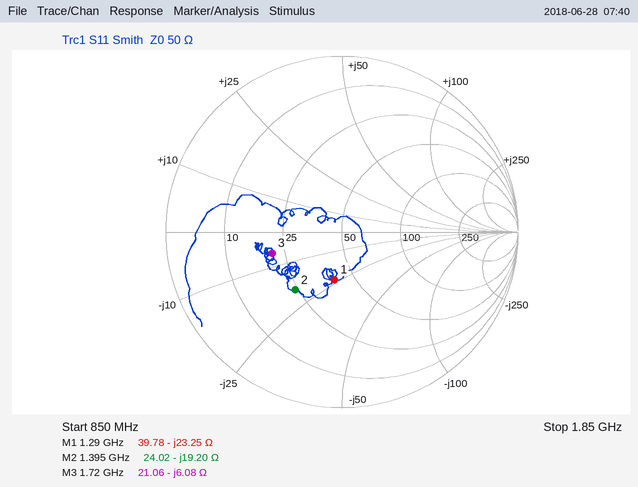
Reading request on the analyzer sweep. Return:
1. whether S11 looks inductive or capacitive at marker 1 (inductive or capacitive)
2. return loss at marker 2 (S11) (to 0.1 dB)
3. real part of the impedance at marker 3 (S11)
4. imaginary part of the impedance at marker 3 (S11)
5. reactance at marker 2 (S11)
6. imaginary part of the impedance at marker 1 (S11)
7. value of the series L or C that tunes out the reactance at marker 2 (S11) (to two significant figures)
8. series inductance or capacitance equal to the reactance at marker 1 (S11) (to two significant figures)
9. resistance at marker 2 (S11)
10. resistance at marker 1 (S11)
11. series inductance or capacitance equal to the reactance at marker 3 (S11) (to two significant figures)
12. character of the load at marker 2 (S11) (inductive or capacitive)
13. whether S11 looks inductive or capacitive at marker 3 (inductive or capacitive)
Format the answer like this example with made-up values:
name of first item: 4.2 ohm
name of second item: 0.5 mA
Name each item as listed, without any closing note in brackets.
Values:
whether S11 looks inductive or capacitive at marker 1: capacitive
return loss at marker 2 (S11): 7.5 dB
real part of the impedance at marker 3: 21.06 Ω
imaginary part of the impedance at marker 3: -6.08 Ω
reactance at marker 2: -19.20 Ω
imaginary part of the impedance at marker 1: -23.25 Ω
value of the series L or C that tunes out the reactance at marker 2 (S11): 2.2 nH
series inductance or capacitance equal to the reactance at marker 1 (S11): 5.3 pF
resistance at marker 2: 24.02 Ω
resistance at marker 1: 39.78 Ω
series inductance or capacitance equal to the reactance at marker 3 (S11): 15 pF
character of the load at marker 2 (S11): capacitive
whether S11 looks inductive or capacitive at marker 3: capacitive
